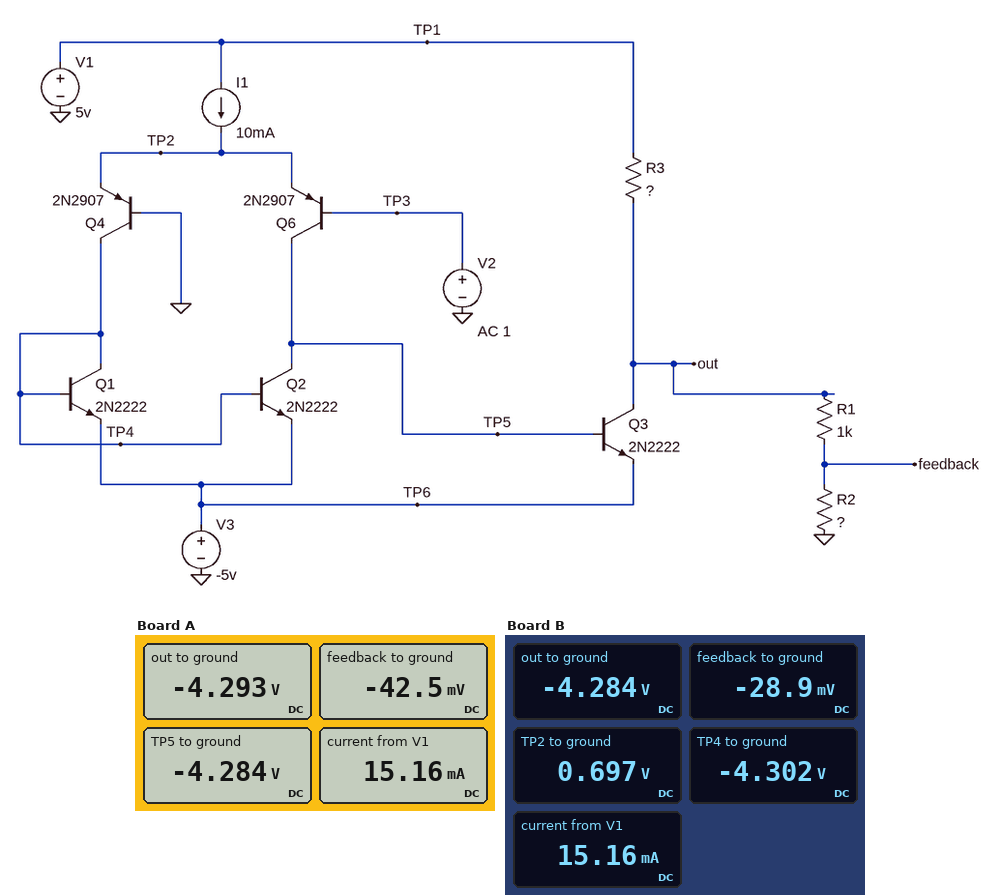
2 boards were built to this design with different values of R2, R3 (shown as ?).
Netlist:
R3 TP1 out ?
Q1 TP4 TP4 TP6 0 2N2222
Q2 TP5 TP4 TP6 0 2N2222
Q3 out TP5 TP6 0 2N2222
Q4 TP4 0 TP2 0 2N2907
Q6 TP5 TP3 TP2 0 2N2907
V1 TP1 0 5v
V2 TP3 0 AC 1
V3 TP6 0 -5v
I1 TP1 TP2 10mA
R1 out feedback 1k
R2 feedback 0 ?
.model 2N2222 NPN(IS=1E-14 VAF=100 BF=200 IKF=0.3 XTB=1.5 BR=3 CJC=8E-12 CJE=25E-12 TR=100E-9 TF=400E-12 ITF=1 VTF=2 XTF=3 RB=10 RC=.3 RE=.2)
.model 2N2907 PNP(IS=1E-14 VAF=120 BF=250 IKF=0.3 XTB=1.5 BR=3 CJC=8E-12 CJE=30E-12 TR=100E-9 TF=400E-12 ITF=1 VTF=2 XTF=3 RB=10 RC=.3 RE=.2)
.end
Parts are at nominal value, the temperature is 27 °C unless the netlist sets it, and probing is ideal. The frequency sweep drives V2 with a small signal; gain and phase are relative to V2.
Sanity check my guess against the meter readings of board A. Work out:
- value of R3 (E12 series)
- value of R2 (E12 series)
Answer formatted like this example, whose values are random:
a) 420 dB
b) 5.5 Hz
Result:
a) 1.8 kΩ
b) 10 Ω
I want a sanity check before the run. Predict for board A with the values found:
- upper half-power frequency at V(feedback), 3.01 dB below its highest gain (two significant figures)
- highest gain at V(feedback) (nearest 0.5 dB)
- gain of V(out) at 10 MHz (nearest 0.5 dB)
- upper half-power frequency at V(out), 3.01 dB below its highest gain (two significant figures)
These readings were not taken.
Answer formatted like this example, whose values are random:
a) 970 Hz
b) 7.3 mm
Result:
a) 160 kHz
b) 46.0 dB
c) 50.0 dB
d) 160 kHz
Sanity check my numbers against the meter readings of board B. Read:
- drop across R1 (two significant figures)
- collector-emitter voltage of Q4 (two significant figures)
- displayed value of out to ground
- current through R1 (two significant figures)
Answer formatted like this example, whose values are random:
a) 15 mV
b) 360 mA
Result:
a) 4.3 V
b) -5.0 V
c) -4.284 V
d) 4.3 mA
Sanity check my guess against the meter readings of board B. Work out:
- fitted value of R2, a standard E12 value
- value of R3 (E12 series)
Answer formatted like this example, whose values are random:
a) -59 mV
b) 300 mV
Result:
a) 6.8 Ω
b) 1.8 kΩ
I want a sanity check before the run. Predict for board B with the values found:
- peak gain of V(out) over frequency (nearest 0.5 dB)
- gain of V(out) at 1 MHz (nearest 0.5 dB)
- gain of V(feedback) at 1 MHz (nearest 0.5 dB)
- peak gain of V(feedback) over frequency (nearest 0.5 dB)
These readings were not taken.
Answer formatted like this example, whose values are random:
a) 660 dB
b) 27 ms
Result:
a) 86.0 dB
b) 70.0 dB
c) 26.5 dB
d) 42.5 dB
